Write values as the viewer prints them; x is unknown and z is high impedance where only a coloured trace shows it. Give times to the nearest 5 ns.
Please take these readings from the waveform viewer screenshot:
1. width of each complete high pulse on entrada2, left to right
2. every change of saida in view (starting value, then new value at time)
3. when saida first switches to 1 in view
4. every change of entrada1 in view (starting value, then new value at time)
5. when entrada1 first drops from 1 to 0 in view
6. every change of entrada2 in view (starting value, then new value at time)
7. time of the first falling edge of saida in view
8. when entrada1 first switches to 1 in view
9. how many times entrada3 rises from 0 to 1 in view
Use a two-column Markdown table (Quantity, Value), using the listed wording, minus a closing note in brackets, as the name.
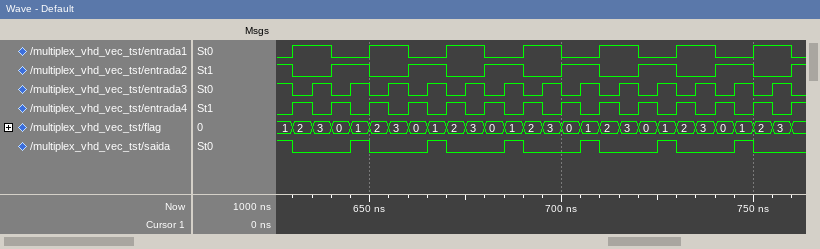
| Quantity | Value |
|---|---|
| width of each complete high pulse on entrada2, left to right | 10 ns, 10 ns, 10 ns, 10 ns, 10 ns, 10 ns |
| every change of saida in view | 1, 0 at 630 ns, 1 at 645 ns, 0 at 650 ns, 1 at 665 ns, 0 at 670 ns, 1 at 685 ns, 0 at 690 ns, 1 at 705 ns, 0 at 710 ns, 1 at 725 ns, 0 at 730 ns, 1 at 745 ns, 0 at 750 ns |
| when saida first switches to 1 in view | 645 ns |
| every change of entrada1 in view | 0, 1 at 630 ns, 0 at 640 ns, 1 at 650 ns, 0 at 660 ns, 1 at 670 ns, 0 at 680 ns, 1 at 690 ns, 0 at 700 ns, 1 at 710 ns, 0 at 720 ns, 1 at 730 ns, 0 at 740 ns, 1 at 750 ns, 0 at 760 ns |
| when entrada1 first drops from 1 to 0 in view | 640 ns |
| every change of entrada2 in view | 1, 0 at 630 ns, 1 at 640 ns, 0 at 650 ns, 1 at 660 ns, 0 at 670 ns, 1 at 680 ns, 0 at 690 ns, 1 at 700 ns, 0 at 710 ns, 1 at 720 ns, 0 at 730 ns, 1 at 740 ns, 0 at 750 ns, 1 at 760 ns |
| time of the first falling edge of saida in view | 630 ns |
| when entrada1 first switches to 1 in view | 630 ns |
| how many times entrada3 rises from 0 to 1 in view | 13 |
